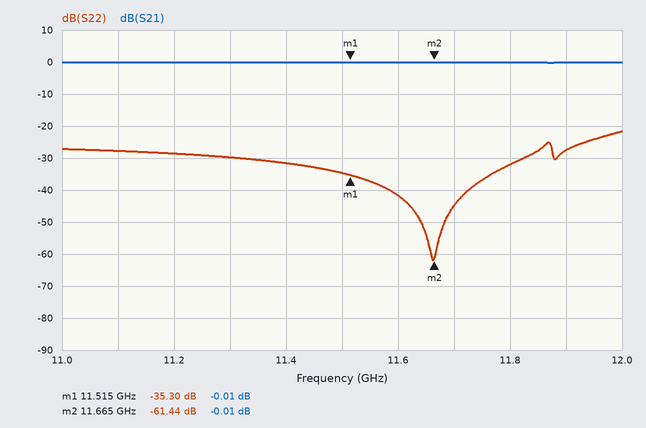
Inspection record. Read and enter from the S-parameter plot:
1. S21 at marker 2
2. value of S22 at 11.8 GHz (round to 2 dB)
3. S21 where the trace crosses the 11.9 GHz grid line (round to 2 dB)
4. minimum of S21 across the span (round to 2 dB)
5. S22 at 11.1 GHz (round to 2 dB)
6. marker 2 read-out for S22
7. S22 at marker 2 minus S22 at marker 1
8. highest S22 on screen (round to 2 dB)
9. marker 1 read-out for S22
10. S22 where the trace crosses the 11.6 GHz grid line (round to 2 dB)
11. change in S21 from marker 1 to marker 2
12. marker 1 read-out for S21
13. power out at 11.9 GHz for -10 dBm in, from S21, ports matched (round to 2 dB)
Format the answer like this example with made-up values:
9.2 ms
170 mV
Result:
-0.01 dB
-32 dB
0 dB
0 dB
-28 dB
-61.44 dB
-26.14 dB
-22 dB
-35.30 dB
-42 dB
0.00 dB
-0.01 dB
-10 dBm
